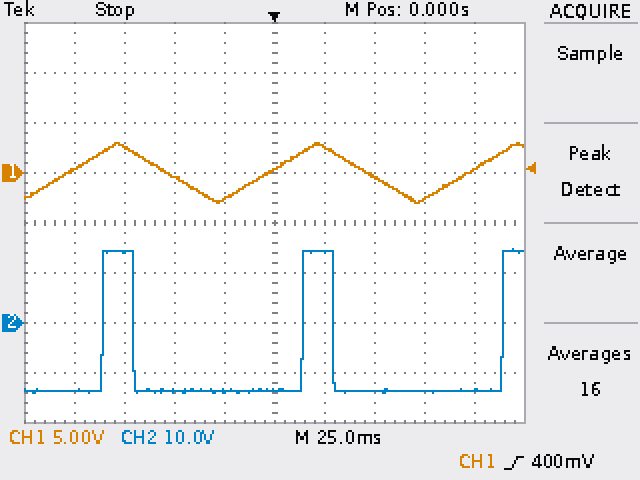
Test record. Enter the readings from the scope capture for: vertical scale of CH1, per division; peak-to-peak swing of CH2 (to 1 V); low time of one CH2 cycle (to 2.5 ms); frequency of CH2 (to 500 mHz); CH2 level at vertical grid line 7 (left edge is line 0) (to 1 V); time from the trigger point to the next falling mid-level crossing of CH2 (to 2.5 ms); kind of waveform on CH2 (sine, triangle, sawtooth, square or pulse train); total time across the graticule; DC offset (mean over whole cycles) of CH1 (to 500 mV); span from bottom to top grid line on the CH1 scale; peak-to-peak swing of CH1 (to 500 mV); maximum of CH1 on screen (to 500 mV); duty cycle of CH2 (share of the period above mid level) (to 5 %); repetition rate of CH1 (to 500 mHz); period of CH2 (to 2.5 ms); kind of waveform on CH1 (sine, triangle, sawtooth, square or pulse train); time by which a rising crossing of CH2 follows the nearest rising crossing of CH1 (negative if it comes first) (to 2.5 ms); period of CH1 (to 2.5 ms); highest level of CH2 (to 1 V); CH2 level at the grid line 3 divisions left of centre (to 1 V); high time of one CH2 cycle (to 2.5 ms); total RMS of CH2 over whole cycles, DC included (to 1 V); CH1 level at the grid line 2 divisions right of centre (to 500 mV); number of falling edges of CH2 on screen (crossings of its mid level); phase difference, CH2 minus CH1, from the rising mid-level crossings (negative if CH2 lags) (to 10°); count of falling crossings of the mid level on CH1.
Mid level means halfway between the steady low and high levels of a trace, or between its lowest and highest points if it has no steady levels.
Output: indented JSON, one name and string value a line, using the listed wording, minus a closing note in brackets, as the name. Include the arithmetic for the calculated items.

{
  "vertical scale of CH1, per division": "5 V",
  "peak-to-peak swing of CH2": "15 V − (-14 V) = 29 V",
  "low time of one CH2 cycle": "85.0 ms",
  "frequency of CH2": "1 / 100.0 ms ≈ 10.0 Hz",
  "CH2 level at vertical grid line 7 (left edge is line 0)": "-14 V",
  "time from the trigger point to the next falling mid-level crossing of CH2": "30.0 ms",
  "kind of waveform on CH2": "pulse train",
  "total time across the graticule": "250 ms",
  "DC offset (mean over whole cycles) of CH1": "(3.0 V + (-3.0 V)) / 2 ≈ 0.0 V",
  "span from bottom to top grid line on the CH1 scale": "40 V",
  "peak-to-peak swing of CH1": "3.0 V − (-3.0 V) = 6.0 V",
  "maximum of CH1 on screen": "3.0 V",
  "duty cycle of CH2 (share of the period above mid level)": "15.0 ms / 100.0 ms ≈ 15 %",
  "repetition rate of CH1": "1 / 100.0 ms ≈ 10.0 Hz",
  "period of CH2": "100.0 ms",
  "kind of waveform on CH1": "triangle",
  "time by which a rising crossing of CH2 follows the nearest rising crossing of CH1 (negative if it comes first)": "+17.5 ms",
  "period of CH1": "100.0 ms",
  "highest level of CH2": "15 V",
  "CH2 level at the grid line 3 divisions left of centre": "14 V",
  "high time of one CH2 cycle": "15.0 ms",
  "total RMS of CH2 over whole cycles, DC included": "√(0.15 × (15 V)² + 0.85 × (-14 V)²) ≈ 14 V",
  "CH1 level at the grid line 2 divisions right of centre": "-500 mV",
  "number of falling edges of CH2 on screen": "2",
  "phase difference, CH2 minus CH1, from the rising mid-level crossings (negative if CH2 lags)": "−360° × (+17.5 ms) / 100.0 ms ≈ -63.0°, so -60° to the nearest 10°",
  "count of falling crossings of the mid level on CH1": "2"
}
